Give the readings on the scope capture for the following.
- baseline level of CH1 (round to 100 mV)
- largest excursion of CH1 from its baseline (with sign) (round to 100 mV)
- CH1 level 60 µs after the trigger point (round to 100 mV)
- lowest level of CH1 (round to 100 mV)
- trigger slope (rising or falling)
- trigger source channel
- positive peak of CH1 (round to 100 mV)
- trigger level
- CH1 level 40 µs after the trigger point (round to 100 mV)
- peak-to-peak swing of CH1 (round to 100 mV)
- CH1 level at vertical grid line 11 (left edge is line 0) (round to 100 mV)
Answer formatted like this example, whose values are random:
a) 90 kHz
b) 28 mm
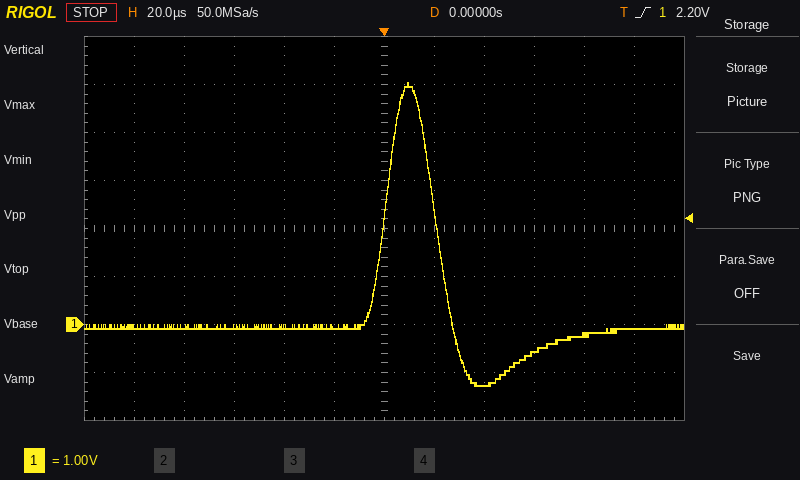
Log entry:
a) -100 mV
b) +5.1 V
c) -600 mV
d) -1.3 V
e) rising
f) CH1
g) 5.0 V
h) 2.20 V
i) -1.3 V
j) 6.3 V
k) -100 mV
